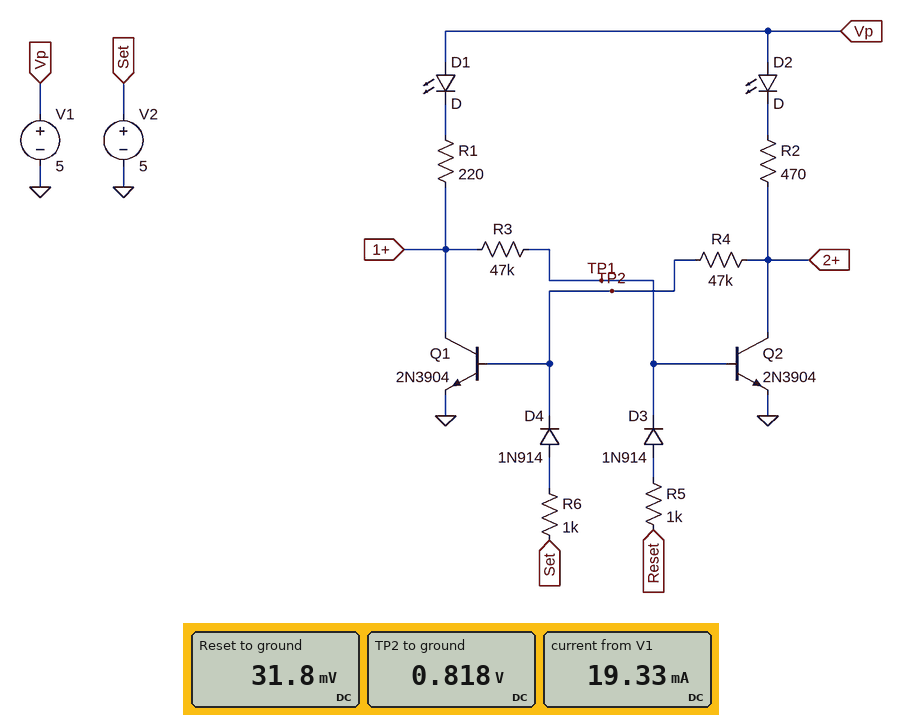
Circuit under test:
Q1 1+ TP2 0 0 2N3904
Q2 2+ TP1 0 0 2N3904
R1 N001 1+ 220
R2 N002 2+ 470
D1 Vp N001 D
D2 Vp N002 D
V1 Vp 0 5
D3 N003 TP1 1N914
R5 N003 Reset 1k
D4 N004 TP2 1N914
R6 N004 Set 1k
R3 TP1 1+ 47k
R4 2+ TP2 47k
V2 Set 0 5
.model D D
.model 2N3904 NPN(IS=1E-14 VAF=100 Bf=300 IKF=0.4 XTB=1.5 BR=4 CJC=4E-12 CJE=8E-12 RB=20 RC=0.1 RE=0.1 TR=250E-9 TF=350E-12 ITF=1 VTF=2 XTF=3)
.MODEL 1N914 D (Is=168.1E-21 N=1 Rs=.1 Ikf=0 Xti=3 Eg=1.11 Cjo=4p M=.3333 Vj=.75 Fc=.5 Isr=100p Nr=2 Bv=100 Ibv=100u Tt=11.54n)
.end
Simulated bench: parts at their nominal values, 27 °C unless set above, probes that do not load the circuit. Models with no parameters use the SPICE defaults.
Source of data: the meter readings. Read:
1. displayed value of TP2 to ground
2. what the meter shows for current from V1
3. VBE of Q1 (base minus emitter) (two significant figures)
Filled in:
0.818 V
19.33 mA
820 mV
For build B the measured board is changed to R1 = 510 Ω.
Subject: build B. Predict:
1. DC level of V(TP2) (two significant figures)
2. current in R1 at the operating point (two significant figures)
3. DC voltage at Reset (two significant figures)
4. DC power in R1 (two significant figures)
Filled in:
810 mV
8.4 mA
19 mV
36 mW
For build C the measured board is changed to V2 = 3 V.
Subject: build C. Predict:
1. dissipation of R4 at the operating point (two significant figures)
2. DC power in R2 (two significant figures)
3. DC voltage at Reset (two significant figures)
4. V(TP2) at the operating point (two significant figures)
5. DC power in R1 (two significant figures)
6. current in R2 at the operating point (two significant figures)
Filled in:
280 µW
2.8 µW
46 mV
770 mV
81 mW
77 µA
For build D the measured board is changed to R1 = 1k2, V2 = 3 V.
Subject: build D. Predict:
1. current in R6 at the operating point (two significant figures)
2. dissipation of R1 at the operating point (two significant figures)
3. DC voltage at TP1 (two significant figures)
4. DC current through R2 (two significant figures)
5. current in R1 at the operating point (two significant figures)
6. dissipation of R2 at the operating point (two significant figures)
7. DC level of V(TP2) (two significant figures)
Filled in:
1.4 mA
15 mW
18 mV
77 µA
3.6 mA
2.8 µW
750 mV
